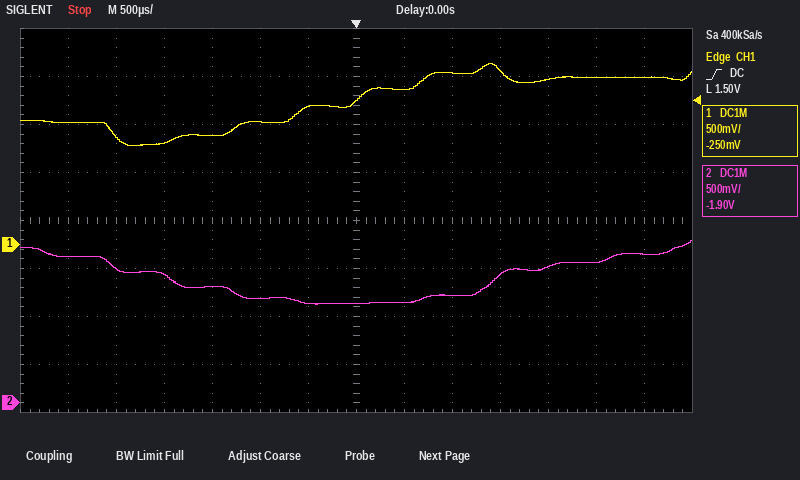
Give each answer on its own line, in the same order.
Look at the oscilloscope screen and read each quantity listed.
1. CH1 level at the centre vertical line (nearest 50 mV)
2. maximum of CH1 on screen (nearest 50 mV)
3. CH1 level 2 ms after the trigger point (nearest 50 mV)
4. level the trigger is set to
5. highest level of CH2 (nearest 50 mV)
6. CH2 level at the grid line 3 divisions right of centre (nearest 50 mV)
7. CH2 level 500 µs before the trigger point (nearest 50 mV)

1.50 V
1.90 V
1.70 V
1.50 V
1.70 V
1.35 V
1.05 V
